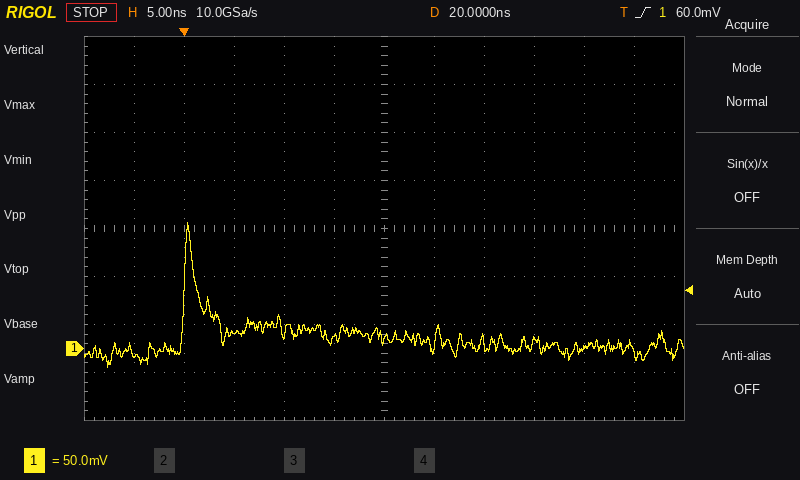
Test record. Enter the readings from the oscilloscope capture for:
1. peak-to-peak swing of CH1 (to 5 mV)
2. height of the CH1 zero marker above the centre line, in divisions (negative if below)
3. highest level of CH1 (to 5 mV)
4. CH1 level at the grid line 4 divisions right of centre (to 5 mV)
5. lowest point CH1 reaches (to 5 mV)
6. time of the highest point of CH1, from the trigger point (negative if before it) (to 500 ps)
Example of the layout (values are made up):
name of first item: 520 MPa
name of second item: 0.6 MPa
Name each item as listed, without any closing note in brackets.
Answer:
peak-to-peak swing of CH1: 150 mV
height of the CH1 zero marker above the centre line, in divisions: -2.5 div
highest level of CH1: 130 mV
CH1 level at the grid line 4 divisions right of centre: 0 mV
lowest point CH1 reaches: -20 mV
time of the highest point of CH1, from the trigger point (negative if before it): +500 ps
